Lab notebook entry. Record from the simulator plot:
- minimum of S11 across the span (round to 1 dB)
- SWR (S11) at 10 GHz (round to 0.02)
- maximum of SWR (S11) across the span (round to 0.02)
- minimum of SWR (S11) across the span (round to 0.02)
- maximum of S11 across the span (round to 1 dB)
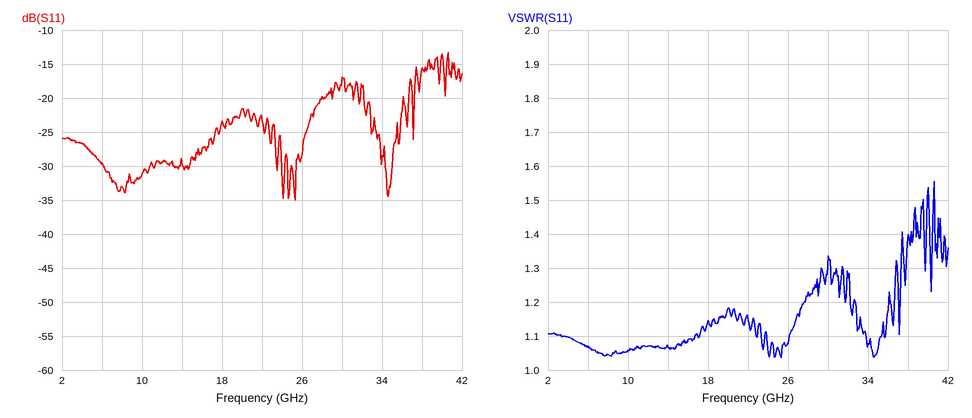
-35 dB
1.06
1.56
1.04
-13 dB
